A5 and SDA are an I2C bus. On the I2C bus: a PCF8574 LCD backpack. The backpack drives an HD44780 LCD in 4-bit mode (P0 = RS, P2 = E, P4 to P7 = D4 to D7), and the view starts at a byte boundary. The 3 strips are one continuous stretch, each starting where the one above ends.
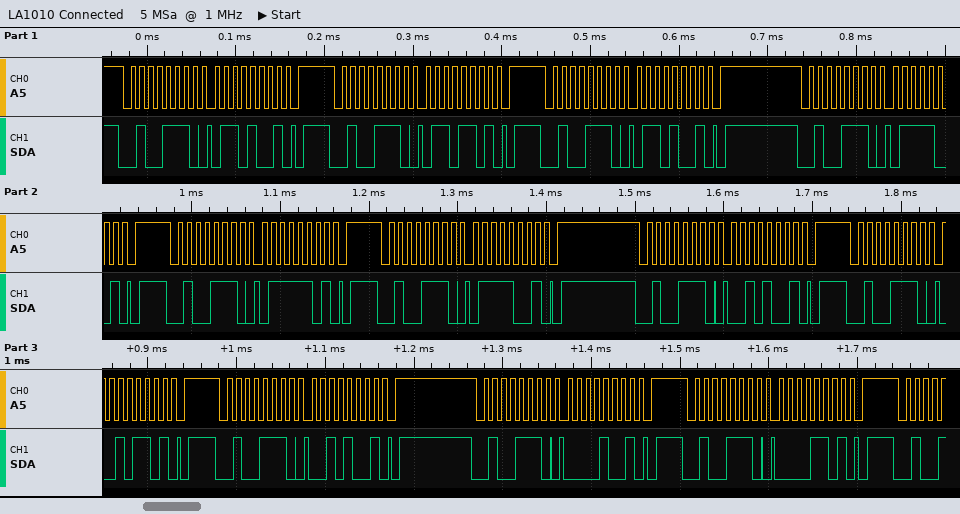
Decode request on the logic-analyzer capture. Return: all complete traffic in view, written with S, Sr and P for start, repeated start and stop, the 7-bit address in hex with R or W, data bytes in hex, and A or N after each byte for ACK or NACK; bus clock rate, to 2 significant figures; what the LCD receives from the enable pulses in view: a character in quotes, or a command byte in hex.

S 27W A 69 A P S 27W A 6D A P S 27W A 69 A P S 27W A 79 A P S 27W A 7D A P S 27W A 79 A P S 27W A 29 A P S 27W A 2D A P S 27W A 29 A P S 27W A 09 A P S 27W A 0D A P
100 kHz
'g'
